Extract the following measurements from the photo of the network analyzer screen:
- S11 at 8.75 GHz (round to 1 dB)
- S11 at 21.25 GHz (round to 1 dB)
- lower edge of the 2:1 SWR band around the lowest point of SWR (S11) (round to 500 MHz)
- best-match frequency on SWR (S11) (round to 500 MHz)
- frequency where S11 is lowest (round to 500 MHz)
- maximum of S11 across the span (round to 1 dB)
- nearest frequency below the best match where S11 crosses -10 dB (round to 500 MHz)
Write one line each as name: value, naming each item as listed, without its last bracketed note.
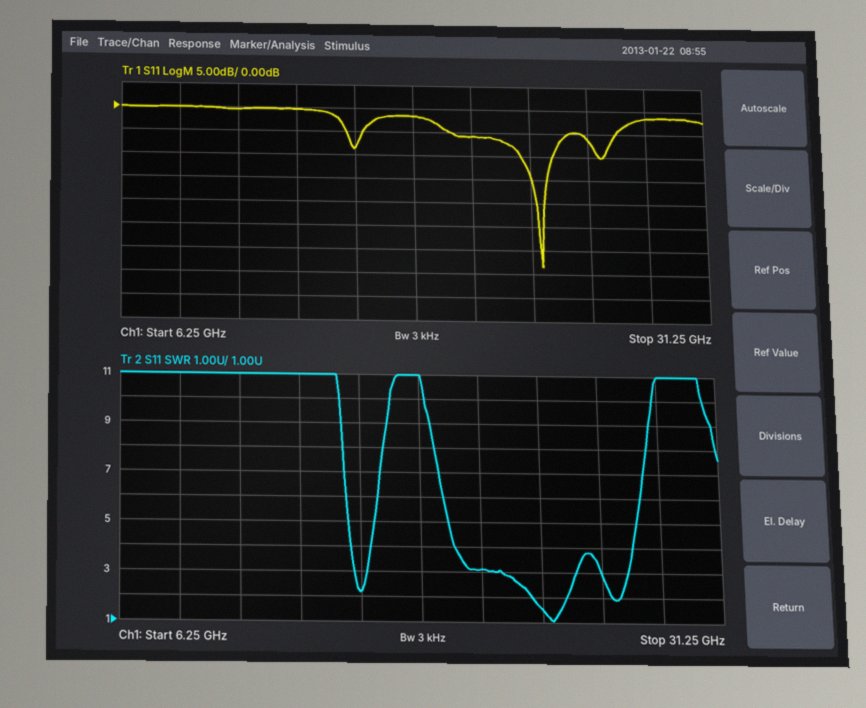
S11 at 8.75 GHz: 0 dB
S11 at 21.25 GHz: -6 dB
lower edge of the 2:1 SWR band around the lowest point of SWR (S11): 23.5 GHz
best-match frequency on SWR (S11): 24.0 GHz
frequency where S11 is lowest: 24.0 GHz
maximum of S11 across the span: 0 dB
nearest frequency below the best match where S11 crosses -10 dB: 23.5 GHz
